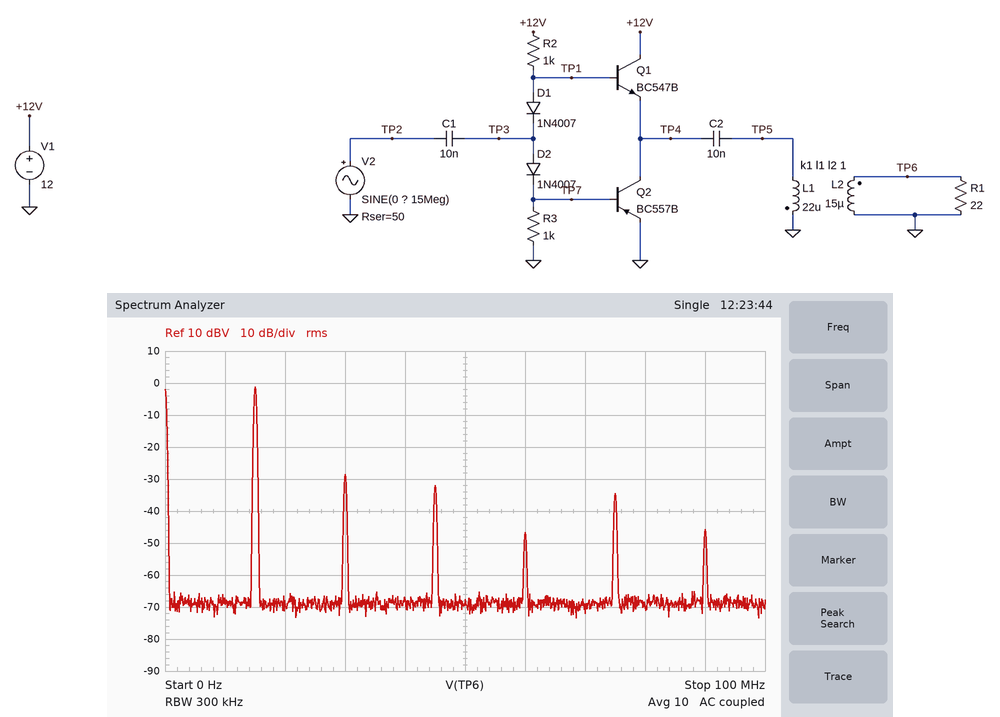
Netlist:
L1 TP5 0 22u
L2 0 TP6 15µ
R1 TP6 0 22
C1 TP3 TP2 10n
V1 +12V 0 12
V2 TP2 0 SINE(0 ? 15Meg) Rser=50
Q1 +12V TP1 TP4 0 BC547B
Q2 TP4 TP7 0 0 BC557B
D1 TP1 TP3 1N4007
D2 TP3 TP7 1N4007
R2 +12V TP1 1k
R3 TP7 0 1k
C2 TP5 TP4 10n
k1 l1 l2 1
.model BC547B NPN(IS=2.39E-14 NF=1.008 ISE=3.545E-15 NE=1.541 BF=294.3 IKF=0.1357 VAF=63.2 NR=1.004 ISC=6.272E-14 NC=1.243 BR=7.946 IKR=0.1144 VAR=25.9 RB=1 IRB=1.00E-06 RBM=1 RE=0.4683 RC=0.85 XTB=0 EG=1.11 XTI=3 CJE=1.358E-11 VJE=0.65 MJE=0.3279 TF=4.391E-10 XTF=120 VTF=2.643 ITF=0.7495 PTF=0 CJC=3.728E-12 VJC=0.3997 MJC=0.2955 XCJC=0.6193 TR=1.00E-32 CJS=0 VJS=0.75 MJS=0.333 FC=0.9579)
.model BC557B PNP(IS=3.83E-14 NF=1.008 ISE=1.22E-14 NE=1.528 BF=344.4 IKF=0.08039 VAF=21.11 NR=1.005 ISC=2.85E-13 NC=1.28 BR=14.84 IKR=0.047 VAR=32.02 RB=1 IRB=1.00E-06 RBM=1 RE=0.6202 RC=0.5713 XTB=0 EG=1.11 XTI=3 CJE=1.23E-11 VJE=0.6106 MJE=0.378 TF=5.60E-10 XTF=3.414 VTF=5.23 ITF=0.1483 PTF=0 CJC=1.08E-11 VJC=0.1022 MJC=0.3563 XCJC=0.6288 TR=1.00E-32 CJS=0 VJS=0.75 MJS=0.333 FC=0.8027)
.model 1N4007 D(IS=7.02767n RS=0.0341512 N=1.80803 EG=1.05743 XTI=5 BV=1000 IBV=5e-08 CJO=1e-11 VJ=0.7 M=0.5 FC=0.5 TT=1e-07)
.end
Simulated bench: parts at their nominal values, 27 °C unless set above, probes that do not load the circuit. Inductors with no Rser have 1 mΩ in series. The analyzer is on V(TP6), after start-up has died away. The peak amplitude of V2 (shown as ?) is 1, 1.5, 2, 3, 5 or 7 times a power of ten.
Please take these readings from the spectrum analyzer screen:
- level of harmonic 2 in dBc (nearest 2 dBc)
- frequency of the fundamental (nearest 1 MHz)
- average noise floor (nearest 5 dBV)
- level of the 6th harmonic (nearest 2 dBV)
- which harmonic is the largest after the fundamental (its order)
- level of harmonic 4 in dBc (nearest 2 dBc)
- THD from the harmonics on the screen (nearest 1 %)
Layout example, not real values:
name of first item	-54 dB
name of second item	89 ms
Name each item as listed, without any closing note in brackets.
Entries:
level of harmonic 2 in dBc	-28 dBc
frequency of the fundamental	15 MHz
average noise floor	-70 dBV
level of the 6th harmonic	-46 dBV
which harmonic is the largest after the fundamental	2
level of harmonic 4 in dBc	-46 dBc
THD from the harmonics on the screen	6 %
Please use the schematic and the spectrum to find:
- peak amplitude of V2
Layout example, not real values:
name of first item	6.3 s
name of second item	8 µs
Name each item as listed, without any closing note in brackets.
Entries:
peak amplitude of V2	2 V
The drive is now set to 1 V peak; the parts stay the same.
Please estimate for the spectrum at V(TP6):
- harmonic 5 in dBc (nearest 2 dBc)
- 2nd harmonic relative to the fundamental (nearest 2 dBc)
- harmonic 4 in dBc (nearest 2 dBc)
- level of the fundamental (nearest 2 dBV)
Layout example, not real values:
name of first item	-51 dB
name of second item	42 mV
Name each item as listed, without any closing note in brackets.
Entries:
harmonic 5 in dBc	-34 dBc
2nd harmonic relative to the fundamental	-30 dBc
harmonic 4 in dBc	-44 dBc
level of the fundamental	-8 dBV
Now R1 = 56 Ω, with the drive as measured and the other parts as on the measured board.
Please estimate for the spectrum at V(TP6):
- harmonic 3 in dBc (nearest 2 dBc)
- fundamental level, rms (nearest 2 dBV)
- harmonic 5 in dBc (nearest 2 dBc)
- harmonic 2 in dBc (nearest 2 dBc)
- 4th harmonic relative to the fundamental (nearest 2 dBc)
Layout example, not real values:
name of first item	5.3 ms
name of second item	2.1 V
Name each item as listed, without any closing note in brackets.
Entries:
harmonic 3 in dBc	-34 dBc
fundamental level, rms	0 dBV
harmonic 5 in dBc	-40 dBc
harmonic 2 in dBc	-38 dBc
4th harmonic relative to the fundamental	-54 dBc
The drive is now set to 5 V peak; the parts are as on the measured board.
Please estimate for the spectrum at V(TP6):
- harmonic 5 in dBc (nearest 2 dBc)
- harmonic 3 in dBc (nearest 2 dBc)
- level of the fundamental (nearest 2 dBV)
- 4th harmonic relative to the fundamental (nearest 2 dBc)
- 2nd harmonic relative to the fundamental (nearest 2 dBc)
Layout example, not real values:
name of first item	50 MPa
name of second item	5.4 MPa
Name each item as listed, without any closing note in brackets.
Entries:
harmonic 5 in dBc	-36 dBc
harmonic 3 in dBc	-26 dBc
level of the fundamental	6 dBV
4th harmonic relative to the fundamental	-30 dBc
2nd harmonic relative to the fundamental	-20 dBc
